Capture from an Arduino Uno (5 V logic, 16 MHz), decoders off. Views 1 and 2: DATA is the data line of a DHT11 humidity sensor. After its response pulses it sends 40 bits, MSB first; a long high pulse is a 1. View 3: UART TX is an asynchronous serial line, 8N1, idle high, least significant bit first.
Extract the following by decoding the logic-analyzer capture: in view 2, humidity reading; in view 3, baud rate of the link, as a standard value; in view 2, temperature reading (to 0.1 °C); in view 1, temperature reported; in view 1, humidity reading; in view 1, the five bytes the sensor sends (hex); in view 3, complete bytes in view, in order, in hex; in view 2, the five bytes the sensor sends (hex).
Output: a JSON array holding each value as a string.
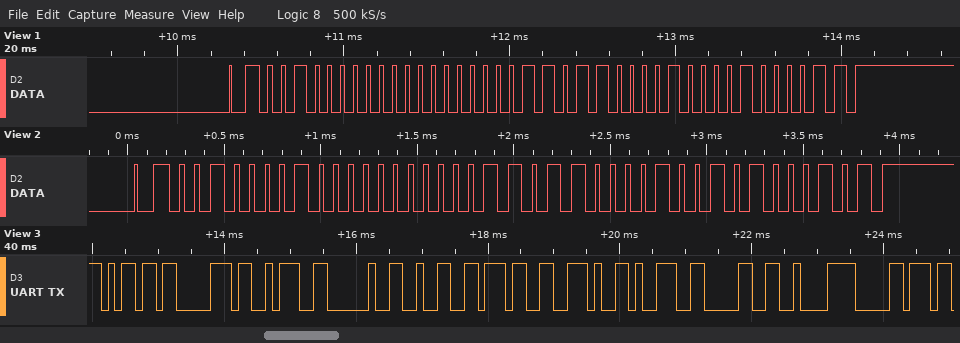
["33 %", "9600 baud", "27.9 °C", "27.8 °C", "32 %", "20 00 1B 08 43", "6D 70 3A 20 32 37 2E 39 30 C2 B0", "21 00 1B 09 45"]
